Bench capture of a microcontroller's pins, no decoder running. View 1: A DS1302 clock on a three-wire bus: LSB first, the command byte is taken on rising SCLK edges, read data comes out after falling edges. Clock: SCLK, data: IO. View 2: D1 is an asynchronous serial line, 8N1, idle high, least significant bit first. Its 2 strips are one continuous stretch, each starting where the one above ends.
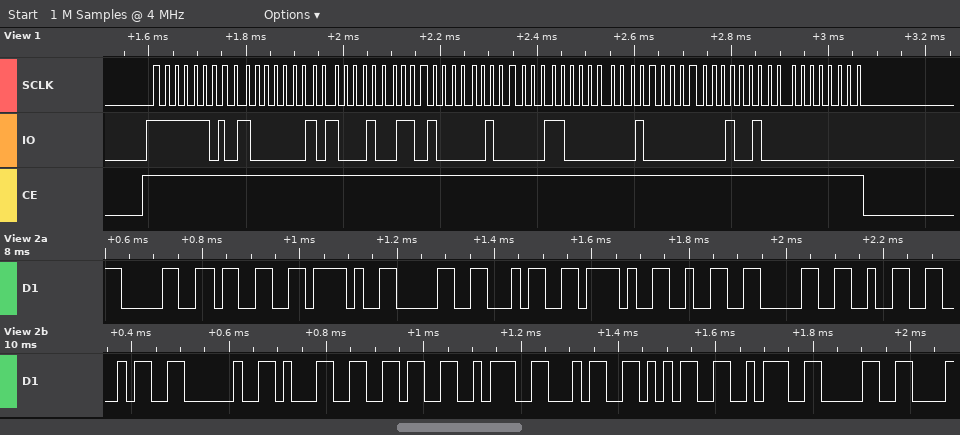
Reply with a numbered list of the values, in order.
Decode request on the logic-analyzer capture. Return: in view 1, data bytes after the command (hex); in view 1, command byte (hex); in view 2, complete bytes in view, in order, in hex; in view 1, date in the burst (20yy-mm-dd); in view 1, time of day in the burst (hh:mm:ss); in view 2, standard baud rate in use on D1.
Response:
1. 02 45 16 04 03 02 24 00
2. 0xBF
3. 30 33 2F 30 34 2F 32 30 32 34 20 31 36 3A 34 35 3A 30
4. 2024-03-04
5. 16:45:02
6. 57600 baud
